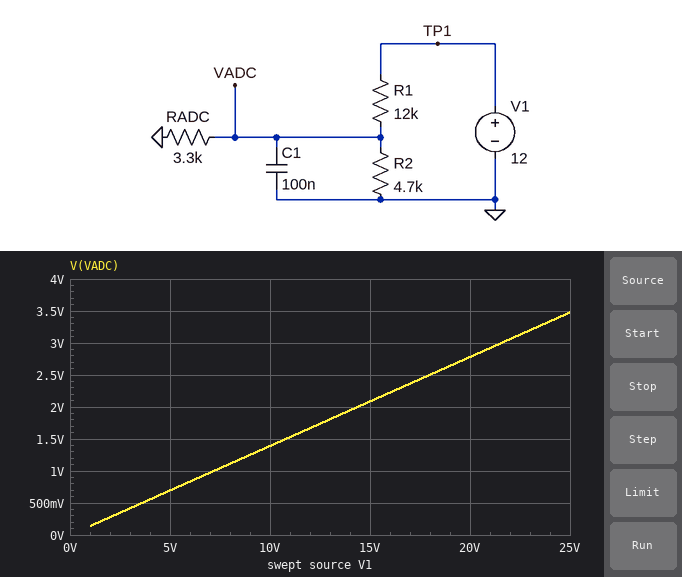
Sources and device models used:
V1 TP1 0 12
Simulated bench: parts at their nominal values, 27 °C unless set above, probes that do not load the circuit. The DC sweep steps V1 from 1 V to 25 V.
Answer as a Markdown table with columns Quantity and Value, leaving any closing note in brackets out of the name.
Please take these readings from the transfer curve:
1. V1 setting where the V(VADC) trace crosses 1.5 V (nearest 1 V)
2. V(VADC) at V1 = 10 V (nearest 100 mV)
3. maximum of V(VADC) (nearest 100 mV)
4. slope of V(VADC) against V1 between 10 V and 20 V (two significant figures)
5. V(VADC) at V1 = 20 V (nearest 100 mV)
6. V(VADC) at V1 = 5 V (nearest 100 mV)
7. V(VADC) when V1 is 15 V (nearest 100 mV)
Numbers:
| Quantity | Value |
|---|---|
| V1 setting where the V(VADC) trace crosses 1.5 V | 11 V |
| V(VADC) at V1 = 10 V | 1.4 V |
| maximum of V(VADC) | 3.5 V |
| slope of V(VADC) against V1 between 10 V and 20 V | 0.14 V/V |
| V(VADC) at V1 = 20 V | 2.8 V |
| V(VADC) at V1 = 5 V | 700 mV |
| V(VADC) when V1 is 15 V | 2.1 V |
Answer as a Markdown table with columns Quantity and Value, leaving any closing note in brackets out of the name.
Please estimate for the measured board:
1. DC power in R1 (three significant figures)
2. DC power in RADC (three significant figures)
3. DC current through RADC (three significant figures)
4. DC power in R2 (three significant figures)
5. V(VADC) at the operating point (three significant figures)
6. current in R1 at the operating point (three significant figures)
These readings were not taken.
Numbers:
| Quantity | Value |
|---|---|
| DC power in R1 | 8.89 mW |
| DC power in RADC | 844 µW |
| DC current through RADC | 506 µA |
| DC power in R2 | 593 µW |
| V(VADC) at the operating point | 1.67 V |
| current in R1 at the operating point | 861 µA |
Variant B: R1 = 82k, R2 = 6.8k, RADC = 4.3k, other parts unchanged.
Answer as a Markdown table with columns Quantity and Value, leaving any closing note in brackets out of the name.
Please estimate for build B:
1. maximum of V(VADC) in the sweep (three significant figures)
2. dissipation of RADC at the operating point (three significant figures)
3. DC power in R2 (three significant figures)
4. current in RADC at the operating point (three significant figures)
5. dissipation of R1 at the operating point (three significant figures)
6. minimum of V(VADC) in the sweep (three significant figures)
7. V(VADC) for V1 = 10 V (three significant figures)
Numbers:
| Quantity | Value |
|---|---|
| maximum of V(VADC) in the sweep | 778 mV |
| dissipation of RADC at the operating point | 32.4 µW |
| DC power in R2 | 20.5 µW |
| current in RADC at the operating point | 86.9 µA |
| dissipation of R1 at the operating point | 1.65 mW |
| minimum of V(VADC) in the sweep | 31.1 mV |
| V(VADC) for V1 = 10 V | 311 mV |
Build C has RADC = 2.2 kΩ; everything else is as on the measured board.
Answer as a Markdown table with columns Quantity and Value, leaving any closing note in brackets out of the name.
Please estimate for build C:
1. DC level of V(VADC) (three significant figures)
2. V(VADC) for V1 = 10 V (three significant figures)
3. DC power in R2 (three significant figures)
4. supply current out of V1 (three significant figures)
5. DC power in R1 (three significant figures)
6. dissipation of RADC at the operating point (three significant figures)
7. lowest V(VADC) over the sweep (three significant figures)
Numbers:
| Quantity | Value |
|---|---|
| DC level of V(VADC) | 1.33 V |
| V(VADC) for V1 = 10 V | 1.11 V |
| DC power in R2 | 378 µW |
| supply current out of V1 | 889 µA |
| DC power in R1 | 9.48 mW |
| dissipation of RADC at the operating point | 807 µW |
| lowest V(VADC) over the sweep | 111 mV |
